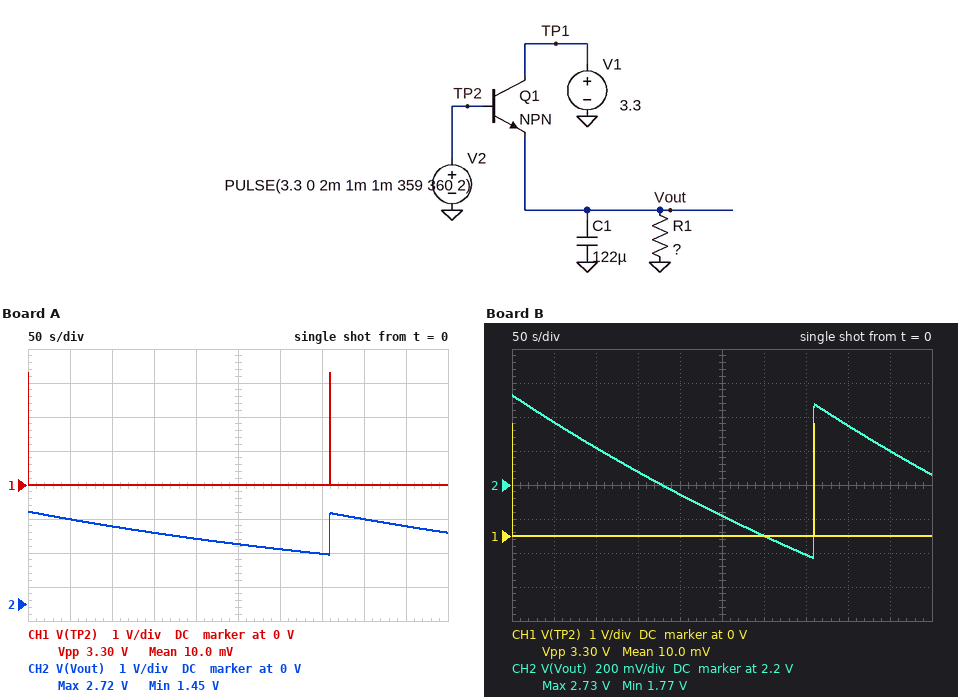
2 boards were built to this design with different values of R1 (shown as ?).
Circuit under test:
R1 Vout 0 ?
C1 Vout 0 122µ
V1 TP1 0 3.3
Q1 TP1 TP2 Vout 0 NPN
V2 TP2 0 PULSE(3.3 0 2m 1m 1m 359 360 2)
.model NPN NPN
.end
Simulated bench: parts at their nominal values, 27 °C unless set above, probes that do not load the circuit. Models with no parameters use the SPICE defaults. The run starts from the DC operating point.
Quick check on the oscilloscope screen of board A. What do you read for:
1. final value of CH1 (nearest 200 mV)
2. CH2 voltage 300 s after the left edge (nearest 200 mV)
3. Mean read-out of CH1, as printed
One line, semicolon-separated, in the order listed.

0 V; 1.6 V; 10.0 mV
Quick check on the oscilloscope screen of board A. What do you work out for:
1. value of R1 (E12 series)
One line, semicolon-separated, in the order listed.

4.7 MΩ
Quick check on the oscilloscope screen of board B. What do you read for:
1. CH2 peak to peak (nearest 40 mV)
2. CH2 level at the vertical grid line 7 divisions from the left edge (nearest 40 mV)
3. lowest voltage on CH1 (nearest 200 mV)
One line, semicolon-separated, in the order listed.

960 mV; 1.80 V; 0 V
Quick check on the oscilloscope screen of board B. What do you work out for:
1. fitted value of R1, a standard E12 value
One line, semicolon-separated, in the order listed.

6.8 MΩ
